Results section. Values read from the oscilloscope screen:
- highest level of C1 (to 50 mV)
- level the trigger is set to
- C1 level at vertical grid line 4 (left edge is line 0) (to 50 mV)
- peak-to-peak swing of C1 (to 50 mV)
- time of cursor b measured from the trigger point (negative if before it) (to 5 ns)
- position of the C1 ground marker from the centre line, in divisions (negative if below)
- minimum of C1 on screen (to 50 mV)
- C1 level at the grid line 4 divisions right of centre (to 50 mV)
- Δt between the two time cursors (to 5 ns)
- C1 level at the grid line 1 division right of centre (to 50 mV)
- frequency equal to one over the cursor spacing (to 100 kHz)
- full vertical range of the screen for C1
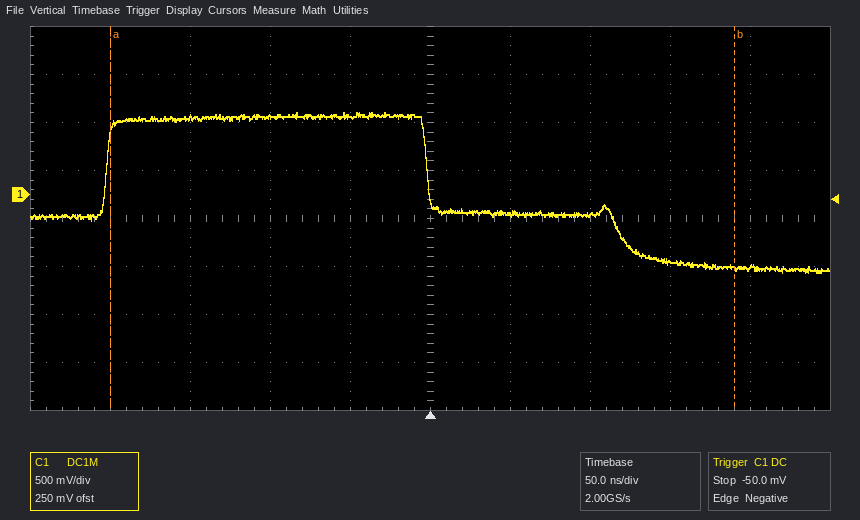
850 mV
-50.0 mV
800 mV
1.65 V
+190 ns
+0.5 div
-800 mV
-750 mV
390 ns
-200 mV
2.6 MHz
4 V
